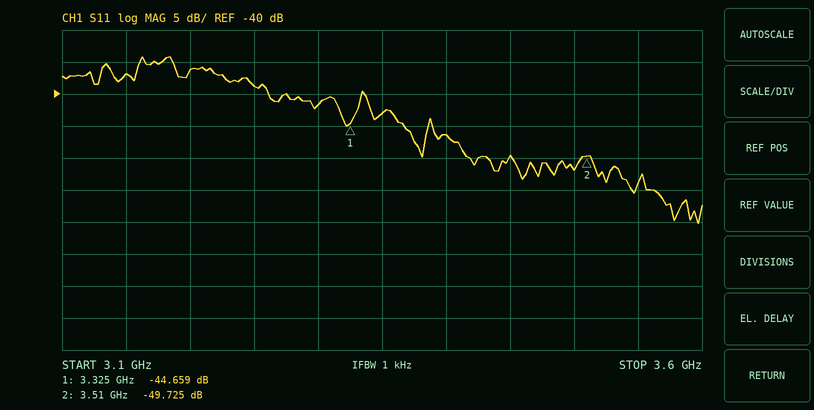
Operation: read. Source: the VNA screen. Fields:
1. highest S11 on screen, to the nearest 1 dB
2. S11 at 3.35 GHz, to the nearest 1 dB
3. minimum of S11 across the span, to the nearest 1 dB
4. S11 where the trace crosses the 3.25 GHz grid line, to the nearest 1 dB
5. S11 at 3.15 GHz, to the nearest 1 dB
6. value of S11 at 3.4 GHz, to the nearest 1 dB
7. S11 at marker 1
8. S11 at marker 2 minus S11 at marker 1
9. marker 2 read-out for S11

-34 dB
-43 dB
-60 dB
-39 dB
-37 dB
-46 dB
-44.659 dB
-5.066 dB
-49.725 dB
